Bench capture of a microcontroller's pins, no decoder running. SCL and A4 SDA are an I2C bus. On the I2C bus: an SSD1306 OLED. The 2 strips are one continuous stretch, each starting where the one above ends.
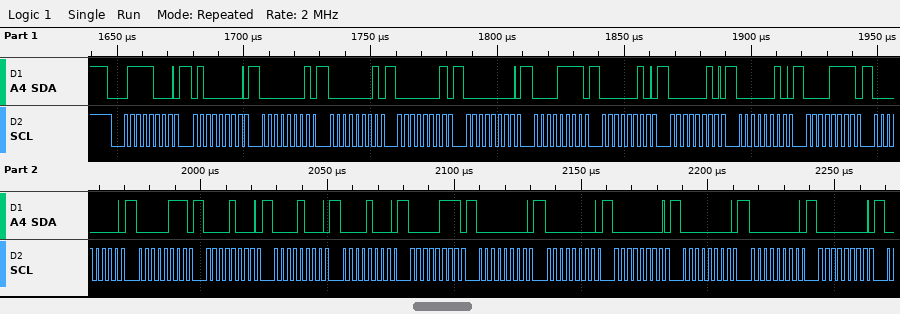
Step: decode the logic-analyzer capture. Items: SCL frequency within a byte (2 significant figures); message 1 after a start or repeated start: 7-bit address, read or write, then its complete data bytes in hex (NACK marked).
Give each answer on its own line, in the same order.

400 kHz
0x3C write: 40 01 01 01 00 0F 02 02 02 0F 00 07 08 08 08 07 00 00 00 00 00 00
